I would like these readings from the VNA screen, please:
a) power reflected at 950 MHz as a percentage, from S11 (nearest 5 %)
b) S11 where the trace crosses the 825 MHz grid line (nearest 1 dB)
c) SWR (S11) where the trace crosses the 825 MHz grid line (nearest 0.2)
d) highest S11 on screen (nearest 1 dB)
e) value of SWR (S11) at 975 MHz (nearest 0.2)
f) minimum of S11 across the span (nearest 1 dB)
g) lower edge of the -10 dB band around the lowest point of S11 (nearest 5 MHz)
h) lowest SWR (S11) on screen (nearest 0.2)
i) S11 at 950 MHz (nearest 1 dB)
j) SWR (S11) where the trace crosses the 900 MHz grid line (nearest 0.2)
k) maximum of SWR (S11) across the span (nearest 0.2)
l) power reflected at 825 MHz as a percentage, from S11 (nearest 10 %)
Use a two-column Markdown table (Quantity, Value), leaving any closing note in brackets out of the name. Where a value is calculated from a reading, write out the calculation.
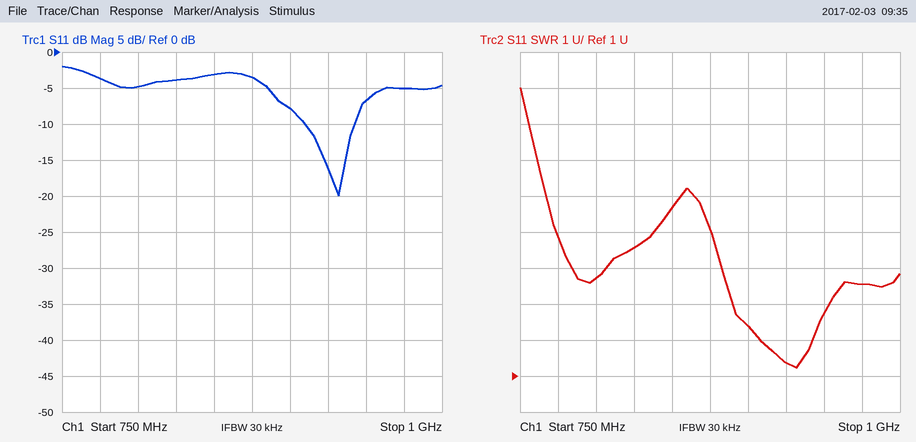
| Quantity | Value |
|---|---|
| power reflected at 950 MHz as a percentage, from S11 | 10^(-7/10) ≈ 20 % |
| S11 where the trace crosses the 825 MHz grid line | -4 dB |
| SWR (S11) where the trace crosses the 825 MHz grid line | 4.6 |
| highest S11 on screen | -2 dB |
| value of SWR (S11) at 975 MHz | 3.6 |
| minimum of S11 across the span | -20 dB |
| lower edge of the -10 dB band around the lowest point of S11 | 910 MHz |
| lowest SWR (S11) on screen | 1.2 |
| S11 at 950 MHz | -7 dB |
| SWR (S11) where the trace crosses the 900 MHz grid line | 2.4 |
| maximum of SWR (S11) across the span | 9.0 |
| power reflected at 825 MHz as a percentage, from S11 | 10^(-4/10) ≈ 40 % |
